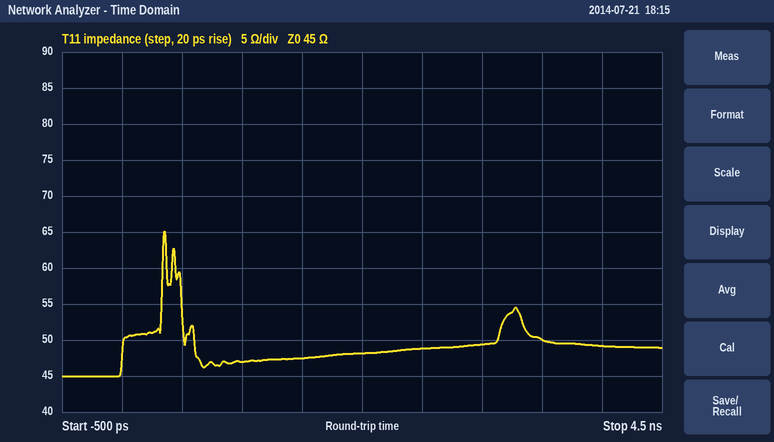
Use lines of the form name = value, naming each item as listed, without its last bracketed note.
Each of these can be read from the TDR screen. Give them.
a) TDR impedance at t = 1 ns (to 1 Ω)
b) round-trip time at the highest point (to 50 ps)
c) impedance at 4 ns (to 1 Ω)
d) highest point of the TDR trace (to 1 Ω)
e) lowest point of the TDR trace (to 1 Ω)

TDR impedance at t = 1 ns = 47 Ω
round-trip time at the highest point = 350 ps
impedance at 4 ns = 49 Ω
highest point of the TDR trace = 65 Ω
lowest point of the TDR trace = 45 Ω
